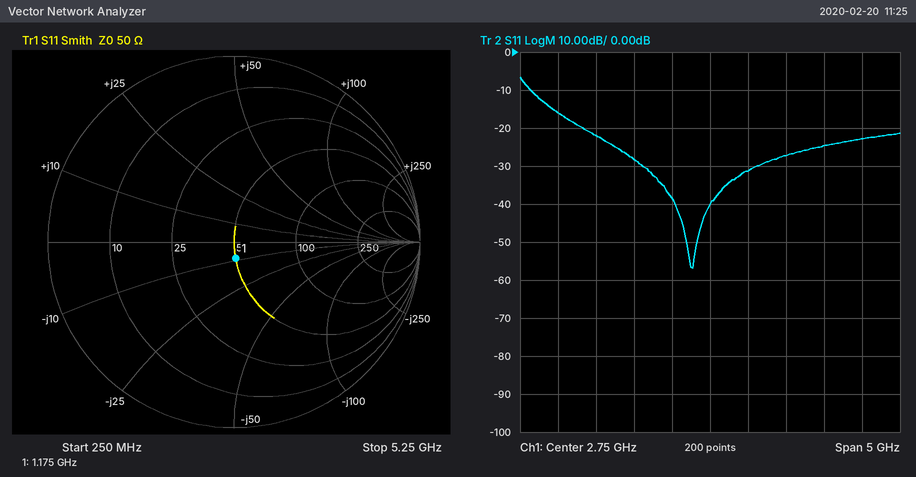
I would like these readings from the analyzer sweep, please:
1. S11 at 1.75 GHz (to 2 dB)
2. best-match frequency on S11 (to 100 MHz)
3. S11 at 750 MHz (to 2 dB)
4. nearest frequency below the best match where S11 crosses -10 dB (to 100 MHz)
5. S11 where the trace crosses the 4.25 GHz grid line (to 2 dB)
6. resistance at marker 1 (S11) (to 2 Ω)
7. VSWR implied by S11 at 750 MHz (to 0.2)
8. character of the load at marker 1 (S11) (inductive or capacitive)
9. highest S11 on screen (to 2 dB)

-28 dB
2.5 GHz
-16 dB
400 MHz
-24 dB
50 Ω
1.4
capacitive
-6 dB
